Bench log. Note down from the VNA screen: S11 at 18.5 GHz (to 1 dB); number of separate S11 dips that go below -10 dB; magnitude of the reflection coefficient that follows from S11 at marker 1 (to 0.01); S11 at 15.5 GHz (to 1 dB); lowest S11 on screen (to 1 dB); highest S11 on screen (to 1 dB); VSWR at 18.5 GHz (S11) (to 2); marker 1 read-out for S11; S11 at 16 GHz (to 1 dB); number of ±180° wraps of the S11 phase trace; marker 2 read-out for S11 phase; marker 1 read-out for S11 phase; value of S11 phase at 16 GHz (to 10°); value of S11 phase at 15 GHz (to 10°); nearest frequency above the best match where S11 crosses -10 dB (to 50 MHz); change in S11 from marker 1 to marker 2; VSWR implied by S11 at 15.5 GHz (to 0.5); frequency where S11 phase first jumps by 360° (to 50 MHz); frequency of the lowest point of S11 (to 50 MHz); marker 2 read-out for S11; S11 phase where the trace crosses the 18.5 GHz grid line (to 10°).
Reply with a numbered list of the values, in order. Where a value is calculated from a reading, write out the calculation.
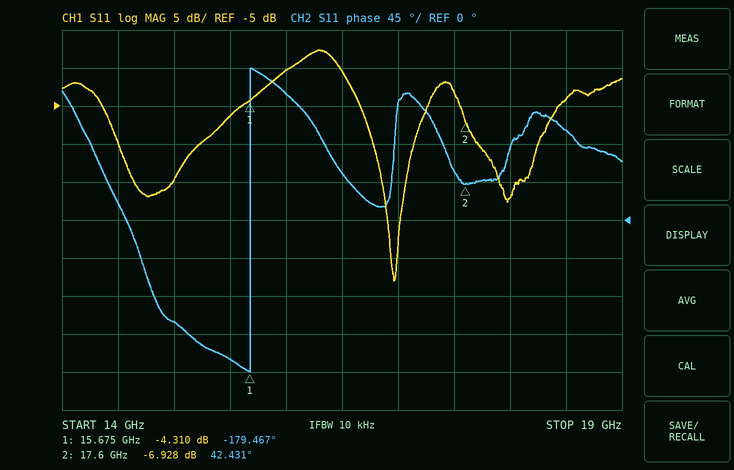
1. -4 dB
2. 3
3. 10^(-4.31/20) ≈ 0.61
4. -6 dB
5. -28 dB
6. 2 dB
7. |Γ| = 10^(-4/20) = 0.6310; VSWR = (1 + 0.6310)/(1 − 0.6310) ≈ 4
8. -4.310 dB
9. 0 dB
10. 1
11. 42.431°
12. -179.467°
13. 150°
14. -120°
15. 17.15 GHz
16. -6.928 − (-4.31) = -2.618 dB
17. |Γ| = 10^(-6/20) = 0.5012; VSWR = (1 + 0.5012)/(1 − 0.5012) ≈ 3.0
18. 15.70 GHz
19. 16.95 GHz
20. -6.928 dB
21. 110°
